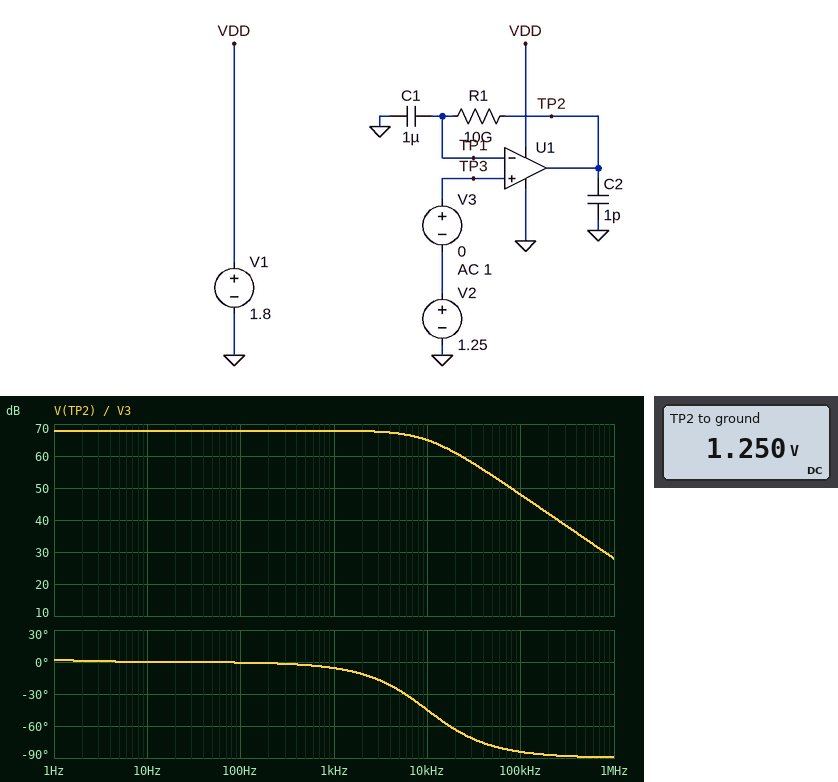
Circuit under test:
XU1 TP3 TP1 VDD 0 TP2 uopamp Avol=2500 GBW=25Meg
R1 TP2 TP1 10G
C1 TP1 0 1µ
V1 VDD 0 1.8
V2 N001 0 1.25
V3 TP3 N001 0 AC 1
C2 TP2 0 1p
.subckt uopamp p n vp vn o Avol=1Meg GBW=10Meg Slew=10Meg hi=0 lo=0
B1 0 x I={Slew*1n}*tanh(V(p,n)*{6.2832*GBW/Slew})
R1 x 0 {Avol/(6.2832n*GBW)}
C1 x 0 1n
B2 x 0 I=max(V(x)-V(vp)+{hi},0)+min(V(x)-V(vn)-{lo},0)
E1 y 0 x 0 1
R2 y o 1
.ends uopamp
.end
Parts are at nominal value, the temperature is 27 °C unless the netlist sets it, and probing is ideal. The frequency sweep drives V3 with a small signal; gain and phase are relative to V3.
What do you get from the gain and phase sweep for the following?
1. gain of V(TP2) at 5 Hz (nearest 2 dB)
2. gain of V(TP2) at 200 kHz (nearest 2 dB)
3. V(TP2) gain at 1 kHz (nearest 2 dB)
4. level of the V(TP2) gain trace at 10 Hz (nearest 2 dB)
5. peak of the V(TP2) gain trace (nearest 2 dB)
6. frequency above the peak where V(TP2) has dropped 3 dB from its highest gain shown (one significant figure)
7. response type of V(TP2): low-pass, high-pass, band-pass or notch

68 dB
42 dB
68 dB
68 dB
68 dB
10 kHz
low-pass
